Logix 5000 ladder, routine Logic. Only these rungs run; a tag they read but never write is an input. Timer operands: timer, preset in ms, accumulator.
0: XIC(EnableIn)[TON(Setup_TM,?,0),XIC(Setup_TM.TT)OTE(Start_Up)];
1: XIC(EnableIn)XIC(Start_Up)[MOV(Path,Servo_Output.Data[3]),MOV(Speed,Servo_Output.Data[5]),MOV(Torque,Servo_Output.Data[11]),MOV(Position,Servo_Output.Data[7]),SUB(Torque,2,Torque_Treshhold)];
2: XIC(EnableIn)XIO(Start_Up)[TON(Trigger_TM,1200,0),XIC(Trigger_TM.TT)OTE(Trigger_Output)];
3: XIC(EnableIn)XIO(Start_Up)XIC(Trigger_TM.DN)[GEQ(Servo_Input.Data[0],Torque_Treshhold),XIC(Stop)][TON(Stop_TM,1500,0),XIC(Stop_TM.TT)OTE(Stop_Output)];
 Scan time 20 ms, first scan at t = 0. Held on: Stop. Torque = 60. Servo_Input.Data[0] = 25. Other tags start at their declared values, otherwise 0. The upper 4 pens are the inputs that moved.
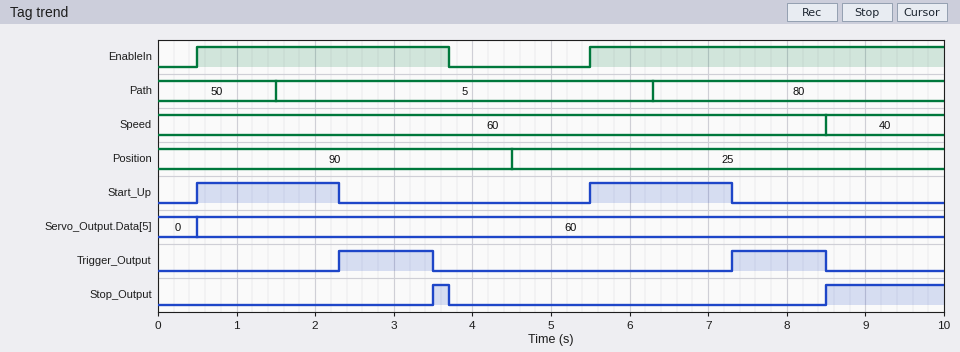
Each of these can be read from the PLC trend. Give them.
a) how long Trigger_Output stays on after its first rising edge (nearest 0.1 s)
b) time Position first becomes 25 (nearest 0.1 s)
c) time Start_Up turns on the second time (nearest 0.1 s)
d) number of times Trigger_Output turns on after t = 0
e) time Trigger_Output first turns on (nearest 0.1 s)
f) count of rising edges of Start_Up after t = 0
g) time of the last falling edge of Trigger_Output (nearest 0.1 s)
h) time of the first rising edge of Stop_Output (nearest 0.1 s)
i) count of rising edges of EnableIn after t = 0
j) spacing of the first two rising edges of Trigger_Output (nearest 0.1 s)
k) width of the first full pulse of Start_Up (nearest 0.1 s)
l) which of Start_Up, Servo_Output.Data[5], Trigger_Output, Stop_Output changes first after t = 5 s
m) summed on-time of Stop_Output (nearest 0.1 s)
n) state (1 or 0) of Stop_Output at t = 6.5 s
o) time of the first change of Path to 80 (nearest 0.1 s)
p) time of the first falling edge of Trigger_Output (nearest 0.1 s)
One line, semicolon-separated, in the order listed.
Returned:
1.2 s; 4.5 s; 5.5 s; 2; 2.3 s; 2; 8.5 s; 3.5 s; 2; 5.0 s; 1.8 s; Start_Up; 1.7 s; 0; 6.3 s; 3.5 s
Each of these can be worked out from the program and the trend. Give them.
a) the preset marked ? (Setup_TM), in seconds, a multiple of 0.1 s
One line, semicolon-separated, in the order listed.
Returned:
1.8 s
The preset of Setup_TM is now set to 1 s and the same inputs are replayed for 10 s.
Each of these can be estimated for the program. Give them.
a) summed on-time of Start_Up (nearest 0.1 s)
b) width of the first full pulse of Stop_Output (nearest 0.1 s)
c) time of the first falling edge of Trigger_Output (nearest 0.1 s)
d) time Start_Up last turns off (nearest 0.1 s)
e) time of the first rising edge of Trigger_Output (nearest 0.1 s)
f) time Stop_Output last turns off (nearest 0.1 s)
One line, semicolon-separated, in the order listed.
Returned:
2.0 s; 1.0 s; 2.7 s; 6.5 s; 1.5 s; 9.2 s
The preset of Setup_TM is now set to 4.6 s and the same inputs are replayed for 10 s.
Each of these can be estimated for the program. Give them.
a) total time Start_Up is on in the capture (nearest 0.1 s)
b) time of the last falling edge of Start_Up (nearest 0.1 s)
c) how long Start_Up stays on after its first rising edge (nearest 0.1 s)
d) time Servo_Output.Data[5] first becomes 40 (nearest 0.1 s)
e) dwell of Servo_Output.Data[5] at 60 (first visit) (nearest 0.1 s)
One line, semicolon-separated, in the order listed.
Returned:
7.7 s; 3.7 s; 3.2 s; 8.5 s; 8.0 s
